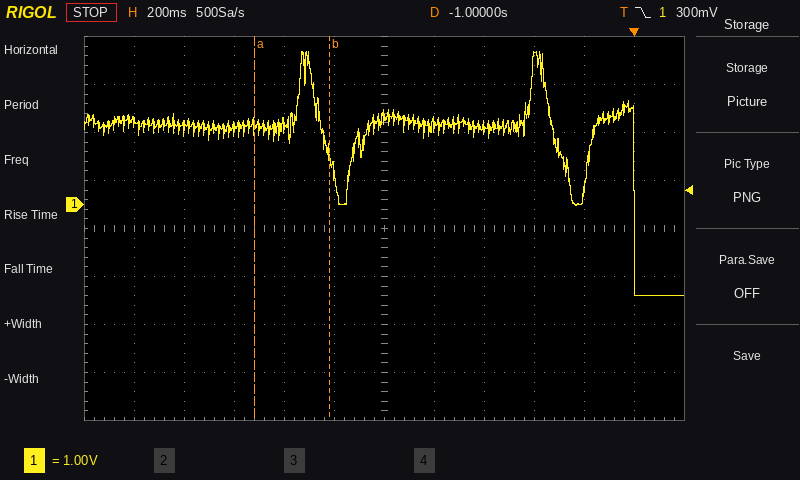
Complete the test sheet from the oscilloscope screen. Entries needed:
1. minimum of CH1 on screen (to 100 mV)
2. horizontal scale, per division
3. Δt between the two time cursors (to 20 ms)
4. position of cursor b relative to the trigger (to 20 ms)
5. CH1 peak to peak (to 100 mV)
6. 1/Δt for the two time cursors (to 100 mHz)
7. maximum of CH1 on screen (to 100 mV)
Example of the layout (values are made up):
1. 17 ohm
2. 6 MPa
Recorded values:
1. -1.9 V
2. 200 ms
3. 300 ms
4. -1.22 s
5. 5.1 V
6. 3.3 Hz
7. 3.2 V
